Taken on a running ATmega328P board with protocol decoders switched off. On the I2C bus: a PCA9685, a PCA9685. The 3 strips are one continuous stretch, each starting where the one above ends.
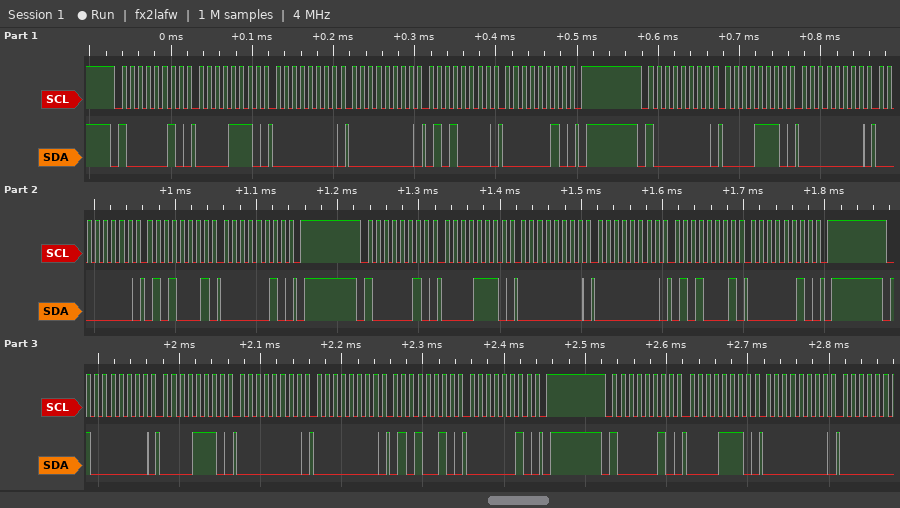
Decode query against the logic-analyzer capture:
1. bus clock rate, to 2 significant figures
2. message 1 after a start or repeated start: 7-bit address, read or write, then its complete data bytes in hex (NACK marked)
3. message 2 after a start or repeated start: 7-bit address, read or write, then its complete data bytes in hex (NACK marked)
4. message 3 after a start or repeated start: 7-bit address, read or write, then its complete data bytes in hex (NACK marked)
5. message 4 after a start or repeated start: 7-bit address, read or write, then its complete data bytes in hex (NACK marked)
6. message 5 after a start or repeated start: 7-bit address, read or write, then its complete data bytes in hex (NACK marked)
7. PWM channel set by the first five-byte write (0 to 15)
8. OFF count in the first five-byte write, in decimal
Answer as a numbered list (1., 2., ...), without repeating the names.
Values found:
1. 100 kHz
2. 0x41 write: 0E 00 00 50 02
3. 0x40 write: 0E 00 00 51 02
4. 0x41 write: 0E 00 00 51 02
5. 0x40 write: 0E 00 00 52 02
6. 0x41 write: 0E 00
7. 2
8. 592
